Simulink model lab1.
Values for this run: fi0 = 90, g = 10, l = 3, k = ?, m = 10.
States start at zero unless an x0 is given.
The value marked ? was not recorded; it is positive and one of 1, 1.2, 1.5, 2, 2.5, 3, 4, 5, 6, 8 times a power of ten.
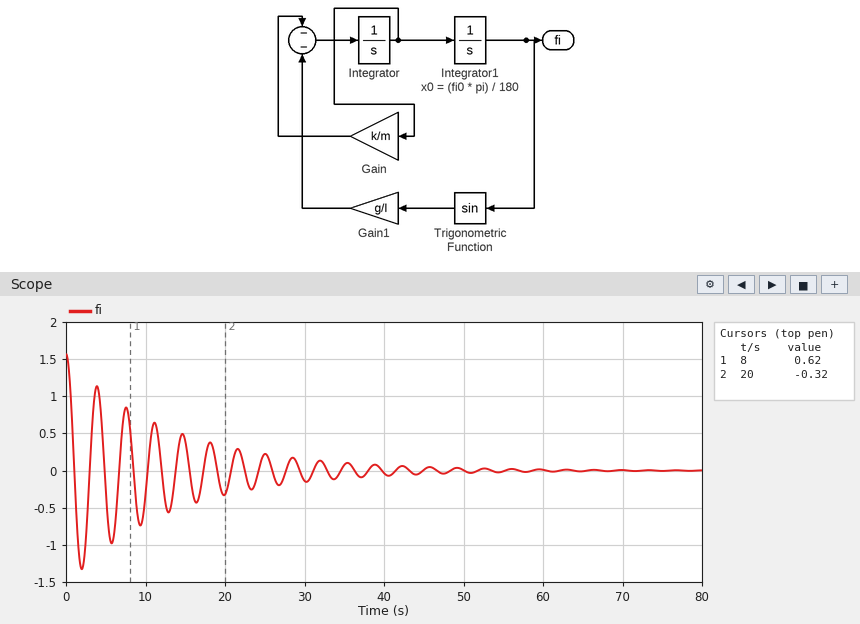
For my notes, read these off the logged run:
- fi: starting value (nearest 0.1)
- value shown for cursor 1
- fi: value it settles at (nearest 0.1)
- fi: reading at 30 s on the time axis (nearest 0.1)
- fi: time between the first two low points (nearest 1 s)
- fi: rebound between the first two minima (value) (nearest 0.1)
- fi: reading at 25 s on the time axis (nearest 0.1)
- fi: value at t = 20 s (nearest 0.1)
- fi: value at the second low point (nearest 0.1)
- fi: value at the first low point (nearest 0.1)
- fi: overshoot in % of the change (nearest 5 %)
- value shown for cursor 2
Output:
1.6
0.62
0.0
-0.1
4 s
1.1
0.2
-0.3
-1.0
-1.3
85 %
-0.32
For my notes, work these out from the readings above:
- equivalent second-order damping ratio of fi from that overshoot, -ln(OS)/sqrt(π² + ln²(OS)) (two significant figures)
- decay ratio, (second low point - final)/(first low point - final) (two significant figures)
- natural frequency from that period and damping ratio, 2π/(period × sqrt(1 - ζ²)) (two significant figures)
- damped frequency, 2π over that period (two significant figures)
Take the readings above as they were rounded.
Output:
0.052
0.77
1.6 rad/s
1.6 rad/s
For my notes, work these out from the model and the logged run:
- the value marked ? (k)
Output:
1.5
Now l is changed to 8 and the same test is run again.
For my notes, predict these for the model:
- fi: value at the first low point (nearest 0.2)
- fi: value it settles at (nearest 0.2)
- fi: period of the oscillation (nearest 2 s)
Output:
-1.2
0.0
6 s
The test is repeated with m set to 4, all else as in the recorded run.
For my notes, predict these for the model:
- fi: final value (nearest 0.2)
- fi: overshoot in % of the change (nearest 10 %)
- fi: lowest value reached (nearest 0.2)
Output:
0.0
70 %
-1.0
